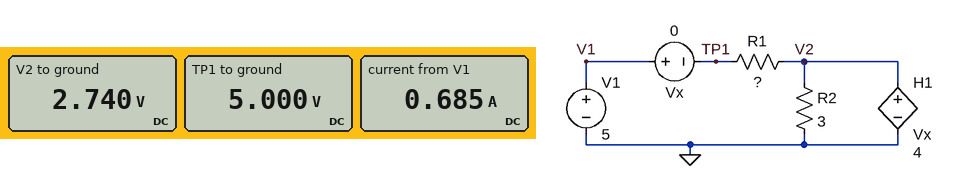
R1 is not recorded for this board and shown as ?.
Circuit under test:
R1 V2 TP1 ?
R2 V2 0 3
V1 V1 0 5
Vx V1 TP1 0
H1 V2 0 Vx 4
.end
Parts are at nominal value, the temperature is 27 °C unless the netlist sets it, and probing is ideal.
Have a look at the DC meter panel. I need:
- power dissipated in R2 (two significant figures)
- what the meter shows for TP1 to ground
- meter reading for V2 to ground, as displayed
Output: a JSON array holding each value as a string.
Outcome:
["2.5 W", "5.000 V", "2.740 V"]
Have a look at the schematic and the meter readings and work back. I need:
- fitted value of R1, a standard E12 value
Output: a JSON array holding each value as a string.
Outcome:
["3.3 Ω"]
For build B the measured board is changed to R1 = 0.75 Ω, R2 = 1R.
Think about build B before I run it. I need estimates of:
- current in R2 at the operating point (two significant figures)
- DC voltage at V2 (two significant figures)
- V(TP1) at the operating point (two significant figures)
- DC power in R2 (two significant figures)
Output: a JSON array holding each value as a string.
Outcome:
["4.2 A", "4.2 V", "5.0 V", "18 W"]
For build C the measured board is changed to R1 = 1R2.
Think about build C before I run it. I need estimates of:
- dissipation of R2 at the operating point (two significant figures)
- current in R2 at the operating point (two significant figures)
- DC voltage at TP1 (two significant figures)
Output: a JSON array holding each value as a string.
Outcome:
["4.9 W", "1.3 A", "5.0 V"]
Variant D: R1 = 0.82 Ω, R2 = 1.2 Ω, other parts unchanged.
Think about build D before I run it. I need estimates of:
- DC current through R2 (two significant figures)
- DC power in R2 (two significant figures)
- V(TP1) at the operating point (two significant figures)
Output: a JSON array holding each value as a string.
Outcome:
["3.5 A", "14 W", "5.0 V"]
